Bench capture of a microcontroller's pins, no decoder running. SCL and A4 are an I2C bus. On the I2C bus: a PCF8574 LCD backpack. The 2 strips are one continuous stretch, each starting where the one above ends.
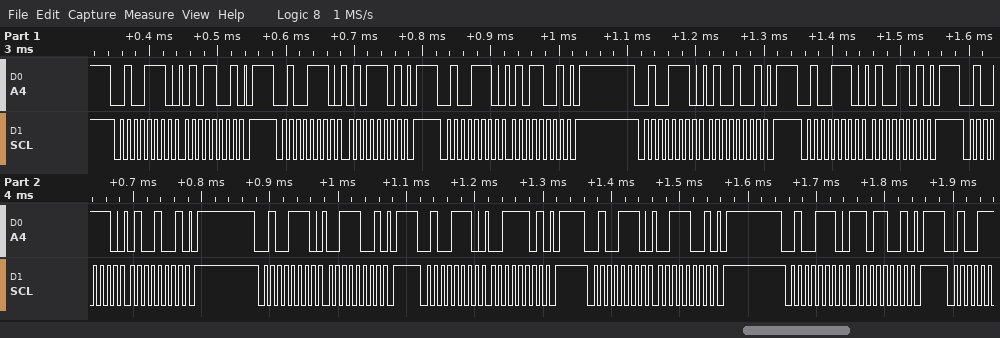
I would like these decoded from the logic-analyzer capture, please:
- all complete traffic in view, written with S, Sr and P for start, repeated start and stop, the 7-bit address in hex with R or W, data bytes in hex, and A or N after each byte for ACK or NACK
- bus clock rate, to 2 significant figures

S 27W A 59 A P S 27W A 5D A P S 27W A 59 A P S 27W A 49 A P S 27W A 4D A P S 27W A 49 A P S 27W A 39 A P S 27W A 3D A P S 27W A 39 A P S 27W A D9 A P
100 kHz
